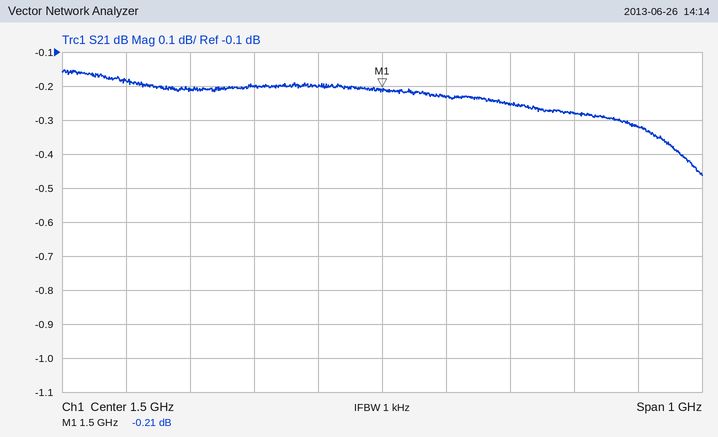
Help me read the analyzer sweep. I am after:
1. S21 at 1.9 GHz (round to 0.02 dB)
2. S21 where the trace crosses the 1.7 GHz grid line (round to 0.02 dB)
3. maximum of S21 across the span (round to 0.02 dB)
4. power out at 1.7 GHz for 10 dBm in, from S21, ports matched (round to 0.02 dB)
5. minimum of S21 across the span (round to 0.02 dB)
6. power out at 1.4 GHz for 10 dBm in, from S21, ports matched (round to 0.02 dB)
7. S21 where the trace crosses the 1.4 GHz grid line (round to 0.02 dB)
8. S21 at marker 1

-0.32 dB
-0.26 dB
-0.16 dB
9.74 dBm
-0.46 dB
9.80 dBm
-0.20 dB
-0.21 dB
